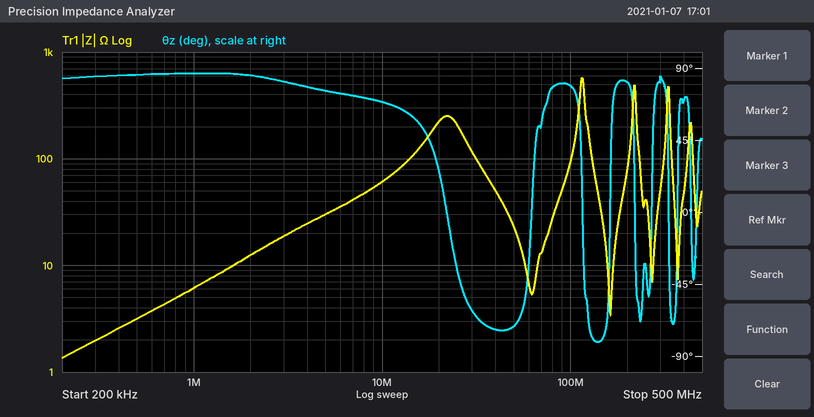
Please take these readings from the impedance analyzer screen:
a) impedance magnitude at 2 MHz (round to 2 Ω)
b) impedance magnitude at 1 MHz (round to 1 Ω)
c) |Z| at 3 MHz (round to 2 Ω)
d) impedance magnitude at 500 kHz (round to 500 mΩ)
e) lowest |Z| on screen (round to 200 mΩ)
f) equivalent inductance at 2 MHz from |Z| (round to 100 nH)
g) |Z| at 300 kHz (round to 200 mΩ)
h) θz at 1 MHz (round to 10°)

12 Ω
6 Ω
18 Ω
3.0 Ω
1.4 Ω
1.0 µH
2.0 Ω
90°
